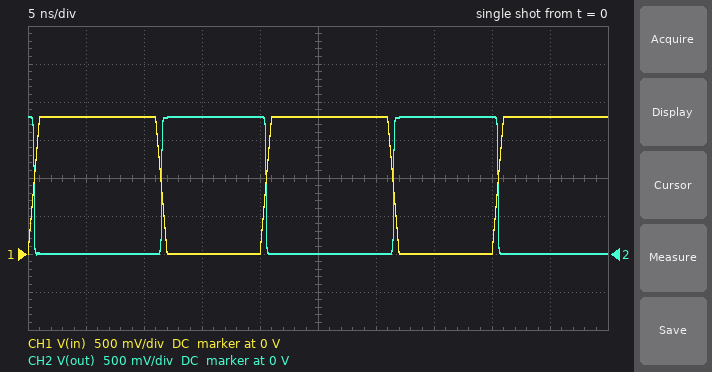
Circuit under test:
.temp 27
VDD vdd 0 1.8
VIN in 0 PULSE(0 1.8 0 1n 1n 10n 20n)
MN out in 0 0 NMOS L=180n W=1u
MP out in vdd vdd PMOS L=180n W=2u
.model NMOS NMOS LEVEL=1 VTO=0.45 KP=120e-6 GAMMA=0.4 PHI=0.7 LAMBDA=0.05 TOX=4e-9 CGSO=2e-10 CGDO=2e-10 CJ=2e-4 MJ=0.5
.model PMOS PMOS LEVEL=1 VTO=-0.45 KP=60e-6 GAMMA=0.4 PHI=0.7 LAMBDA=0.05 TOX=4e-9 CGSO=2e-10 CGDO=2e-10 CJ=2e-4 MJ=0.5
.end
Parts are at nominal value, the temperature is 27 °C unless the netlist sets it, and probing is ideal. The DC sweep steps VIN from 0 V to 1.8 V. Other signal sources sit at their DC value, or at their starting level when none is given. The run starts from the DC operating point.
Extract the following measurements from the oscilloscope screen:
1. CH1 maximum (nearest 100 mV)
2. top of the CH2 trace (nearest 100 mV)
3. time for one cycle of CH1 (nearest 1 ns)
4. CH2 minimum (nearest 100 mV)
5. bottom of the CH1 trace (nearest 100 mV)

1.8 V
1.8 V
20 ns
0 V
0 V
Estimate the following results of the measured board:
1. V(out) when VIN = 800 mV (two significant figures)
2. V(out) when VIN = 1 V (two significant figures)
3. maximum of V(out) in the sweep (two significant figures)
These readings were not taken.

1.7 V
140 mV
1.8 V
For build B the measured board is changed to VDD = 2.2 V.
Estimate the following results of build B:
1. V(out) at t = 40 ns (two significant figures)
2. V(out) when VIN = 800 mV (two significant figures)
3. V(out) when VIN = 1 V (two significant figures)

2.2 V
2.1 V
1.9 V
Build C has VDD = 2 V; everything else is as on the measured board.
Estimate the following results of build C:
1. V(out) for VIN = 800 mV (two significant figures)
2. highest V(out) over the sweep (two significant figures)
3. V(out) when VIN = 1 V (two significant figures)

1.9 V
2.0 V
1.0 V
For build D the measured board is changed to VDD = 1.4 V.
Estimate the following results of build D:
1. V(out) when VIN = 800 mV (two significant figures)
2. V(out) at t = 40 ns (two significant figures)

36 mV
1.4 V
